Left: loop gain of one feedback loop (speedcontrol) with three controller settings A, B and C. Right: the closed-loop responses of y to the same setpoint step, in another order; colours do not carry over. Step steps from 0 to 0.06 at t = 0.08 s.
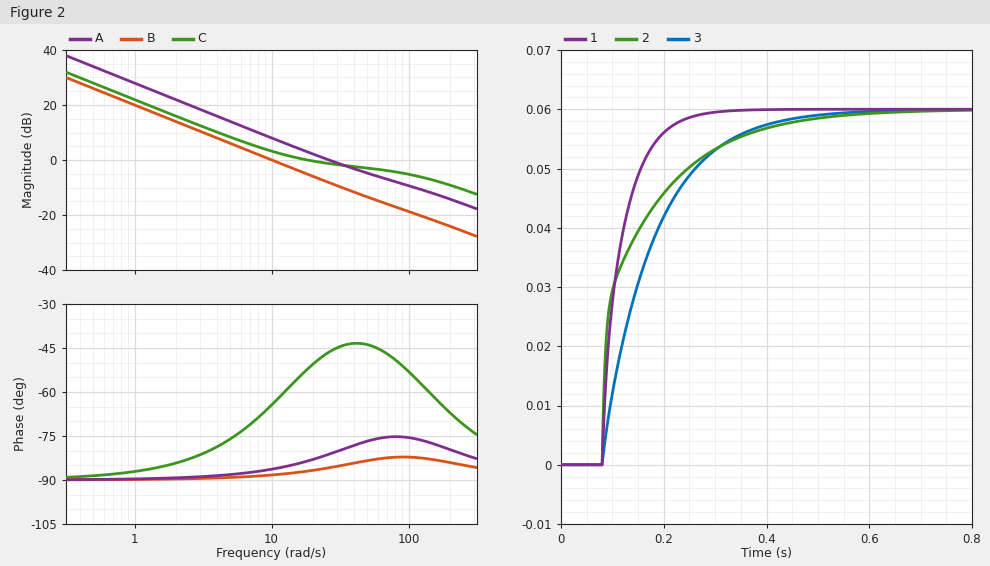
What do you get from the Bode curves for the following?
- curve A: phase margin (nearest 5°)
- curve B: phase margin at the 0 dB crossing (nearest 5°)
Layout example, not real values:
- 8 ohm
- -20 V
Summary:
- 100°
- 90°
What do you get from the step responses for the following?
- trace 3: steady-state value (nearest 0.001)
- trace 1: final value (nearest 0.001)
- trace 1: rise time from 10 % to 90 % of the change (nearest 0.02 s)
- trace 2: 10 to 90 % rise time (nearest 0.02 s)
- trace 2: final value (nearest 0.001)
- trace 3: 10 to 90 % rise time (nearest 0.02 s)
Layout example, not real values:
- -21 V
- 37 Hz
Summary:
- 0.060
- 0.060
- 0.10 s
- 0.24 s
- 0.060
- 0.22 s
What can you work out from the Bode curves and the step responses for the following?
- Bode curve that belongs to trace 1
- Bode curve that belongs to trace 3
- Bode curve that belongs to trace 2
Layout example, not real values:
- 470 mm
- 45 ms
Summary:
- A
- B
- C
